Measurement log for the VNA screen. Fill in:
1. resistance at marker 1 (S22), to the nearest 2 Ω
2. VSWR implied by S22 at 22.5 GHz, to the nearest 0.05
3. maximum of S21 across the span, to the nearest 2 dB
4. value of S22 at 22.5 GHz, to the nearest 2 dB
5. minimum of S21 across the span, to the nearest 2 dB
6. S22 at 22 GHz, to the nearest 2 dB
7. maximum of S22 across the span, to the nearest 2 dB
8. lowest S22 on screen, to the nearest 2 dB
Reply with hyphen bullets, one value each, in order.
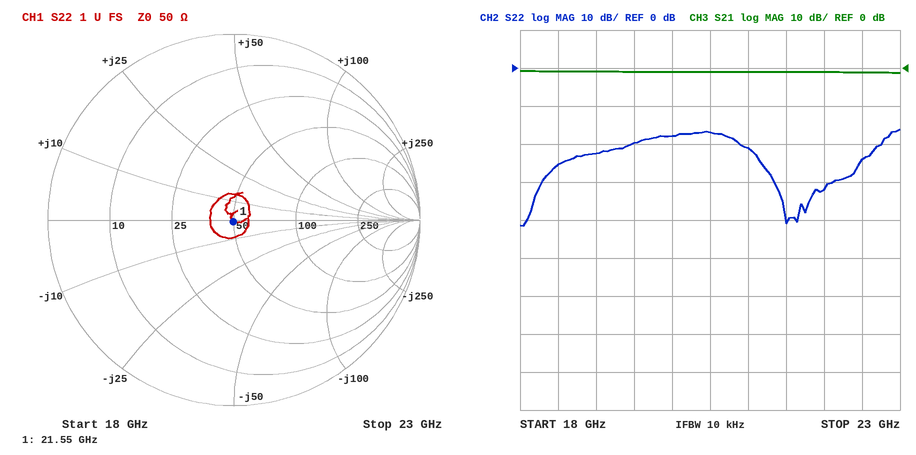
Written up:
- 50 Ω
- 1.15
- 0 dB
- -24 dB
- -2 dB
- -32 dB
- -16 dB
- -42 dB
